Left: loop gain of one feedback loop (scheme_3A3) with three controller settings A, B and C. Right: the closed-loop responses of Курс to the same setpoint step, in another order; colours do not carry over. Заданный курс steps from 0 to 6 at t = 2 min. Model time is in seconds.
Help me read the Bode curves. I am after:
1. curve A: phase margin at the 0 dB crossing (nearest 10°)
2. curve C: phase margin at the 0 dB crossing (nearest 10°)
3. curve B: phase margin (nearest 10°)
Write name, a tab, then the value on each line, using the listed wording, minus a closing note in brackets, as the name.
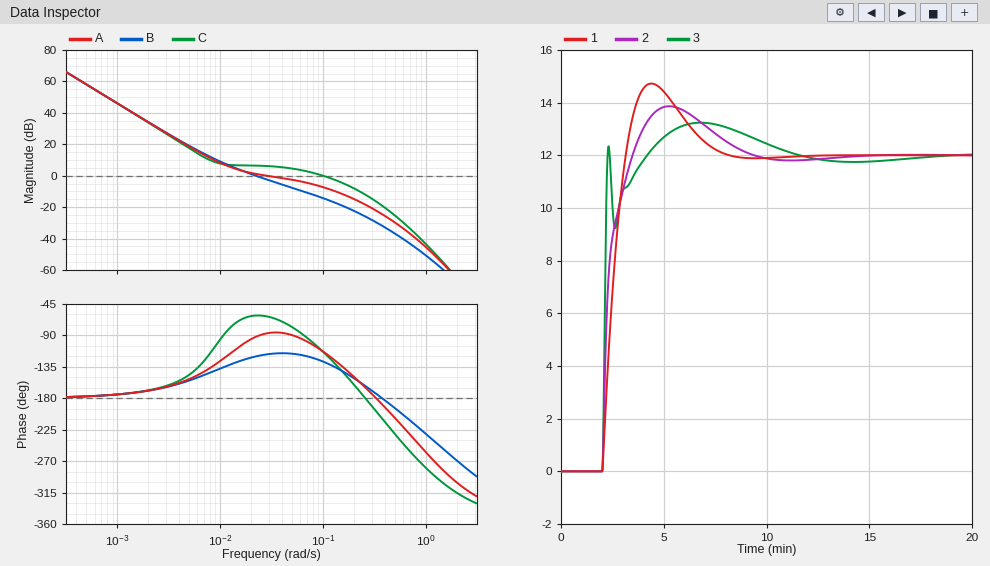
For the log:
curve A: phase margin at the 0 dB crossing	90°
curve C: phase margin at the 0 dB crossing	70°
curve B: phase margin	60°
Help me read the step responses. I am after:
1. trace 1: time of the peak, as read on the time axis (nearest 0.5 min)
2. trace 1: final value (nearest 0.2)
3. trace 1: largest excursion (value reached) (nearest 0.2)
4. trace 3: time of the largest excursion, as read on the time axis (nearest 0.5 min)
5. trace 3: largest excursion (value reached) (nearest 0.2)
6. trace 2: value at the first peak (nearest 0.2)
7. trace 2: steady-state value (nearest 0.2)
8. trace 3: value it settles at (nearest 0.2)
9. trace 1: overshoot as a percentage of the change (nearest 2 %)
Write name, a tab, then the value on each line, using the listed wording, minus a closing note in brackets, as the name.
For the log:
trace 1: time of the peak, as read on the time axis	4.5 min
trace 1: final value	12.0
trace 1: largest excursion (value reached)	14.8
trace 3: time of the largest excursion, as read on the time axis	7.0 min
trace 3: largest excursion (value reached)	13.2
trace 2: value at the first peak	13.8
trace 2: steady-state value	12.0
trace 3: value it settles at	12.0
trace 1: overshoot as a percentage of the change	22 %
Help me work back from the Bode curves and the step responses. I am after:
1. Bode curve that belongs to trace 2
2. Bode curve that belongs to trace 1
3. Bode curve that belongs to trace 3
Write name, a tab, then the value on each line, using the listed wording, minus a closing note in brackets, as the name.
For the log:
Bode curve that belongs to trace 2	A
Bode curve that belongs to trace 1	B
Bode curve that belongs to trace 3	C
